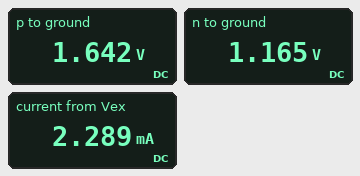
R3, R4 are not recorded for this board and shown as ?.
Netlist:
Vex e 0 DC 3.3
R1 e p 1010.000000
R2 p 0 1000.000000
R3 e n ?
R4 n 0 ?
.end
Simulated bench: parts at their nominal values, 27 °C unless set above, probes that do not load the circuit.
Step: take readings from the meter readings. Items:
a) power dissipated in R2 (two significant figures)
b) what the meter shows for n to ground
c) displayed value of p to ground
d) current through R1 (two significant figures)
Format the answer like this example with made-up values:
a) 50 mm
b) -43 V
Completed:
a) 2.7 mW
b) 1.165 V
c) 1.642 V
d) 1.6 mA
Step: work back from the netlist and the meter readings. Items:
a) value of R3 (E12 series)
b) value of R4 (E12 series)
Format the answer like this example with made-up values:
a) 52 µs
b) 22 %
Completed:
a) 3.3 kΩ
b) 1.8 kΩ
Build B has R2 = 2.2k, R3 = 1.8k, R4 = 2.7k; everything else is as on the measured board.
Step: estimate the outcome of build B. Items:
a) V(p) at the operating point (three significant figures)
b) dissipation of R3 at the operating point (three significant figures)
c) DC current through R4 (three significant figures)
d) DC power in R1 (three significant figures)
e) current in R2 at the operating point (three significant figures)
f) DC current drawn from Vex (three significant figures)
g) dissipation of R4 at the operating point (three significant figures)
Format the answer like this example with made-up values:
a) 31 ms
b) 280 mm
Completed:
a) 2.26 V
b) 968 µW
c) 733 µA
d) 1.07 mW
e) 1.03 mA
f) 1.76 mA
g) 1.45 mW
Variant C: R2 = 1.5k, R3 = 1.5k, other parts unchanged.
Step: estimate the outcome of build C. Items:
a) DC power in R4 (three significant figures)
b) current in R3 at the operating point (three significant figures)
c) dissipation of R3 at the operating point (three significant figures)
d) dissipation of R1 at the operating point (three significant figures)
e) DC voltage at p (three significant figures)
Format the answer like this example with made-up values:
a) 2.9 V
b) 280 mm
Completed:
a) 1.80 mW
b) 1.00 mA
c) 1.50 mW
d) 1.75 mW
e) 1.97 V
